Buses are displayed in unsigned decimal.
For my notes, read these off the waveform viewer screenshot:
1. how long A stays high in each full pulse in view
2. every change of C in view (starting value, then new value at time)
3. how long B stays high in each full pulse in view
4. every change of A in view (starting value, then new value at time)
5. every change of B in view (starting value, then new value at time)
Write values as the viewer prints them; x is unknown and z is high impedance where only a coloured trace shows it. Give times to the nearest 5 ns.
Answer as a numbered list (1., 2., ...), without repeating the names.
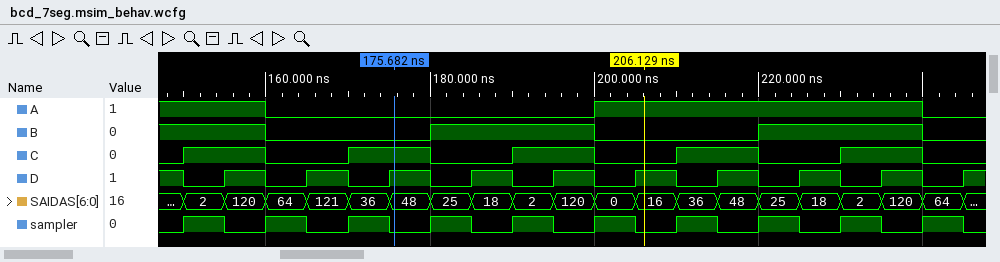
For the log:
1. 40 ns
2. 0, 1 at 150 ns, 0 at 160 ns, 1 at 170 ns, 0 at 180 ns, 1 at 190 ns, 0 at 200 ns, 1 at 210 ns, 0 at 220 ns, 1 at 230 ns, 0 at 240 ns
3. 20 ns, 20 ns
4. 1, 0 at 160 ns, 1 at 200 ns, 0 at 240 ns
5. 1, 0 at 160 ns, 1 at 180 ns, 0 at 200 ns, 1 at 220 ns, 0 at 240 ns
